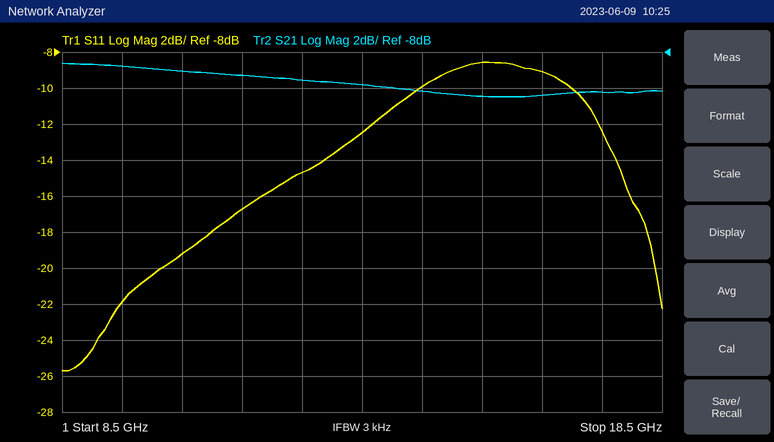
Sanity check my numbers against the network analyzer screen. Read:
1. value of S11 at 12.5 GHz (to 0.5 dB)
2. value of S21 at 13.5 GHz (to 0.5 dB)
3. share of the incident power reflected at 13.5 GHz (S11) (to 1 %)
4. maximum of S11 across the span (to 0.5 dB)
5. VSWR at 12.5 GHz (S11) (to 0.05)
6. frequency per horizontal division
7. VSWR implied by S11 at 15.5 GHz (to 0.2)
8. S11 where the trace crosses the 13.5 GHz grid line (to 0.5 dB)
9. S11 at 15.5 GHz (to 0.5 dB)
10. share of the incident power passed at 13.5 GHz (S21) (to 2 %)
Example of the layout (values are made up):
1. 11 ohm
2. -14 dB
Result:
1. -14.5 dB
2. -10.0 dB
3. 6 %
4. -8.5 dB
5. 1.45
6. 1 GHz
7. 2.2
8. -12.5 dB
9. -8.5 dB
10. 10 %
